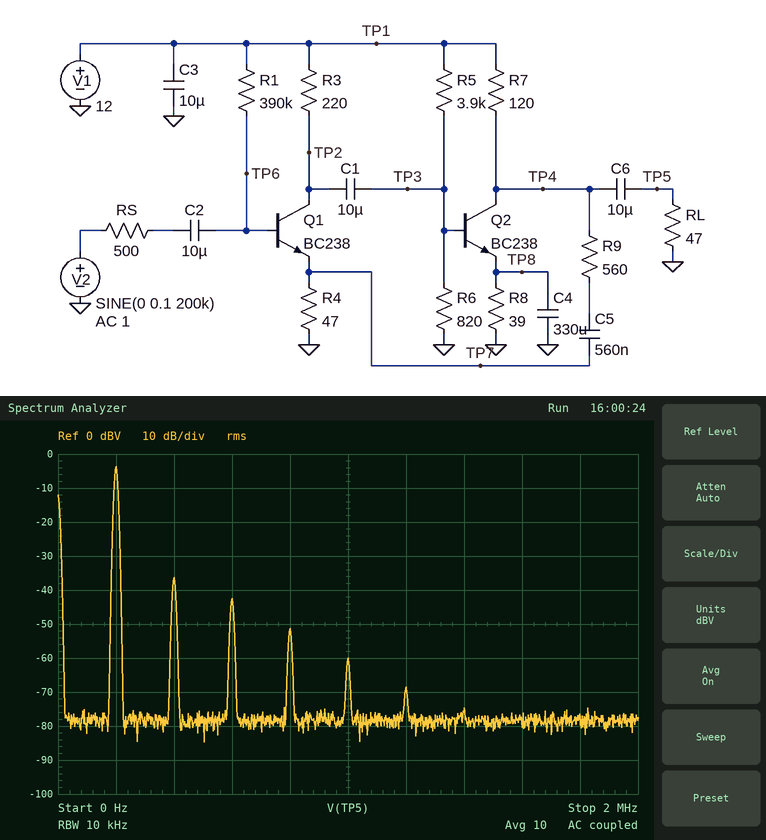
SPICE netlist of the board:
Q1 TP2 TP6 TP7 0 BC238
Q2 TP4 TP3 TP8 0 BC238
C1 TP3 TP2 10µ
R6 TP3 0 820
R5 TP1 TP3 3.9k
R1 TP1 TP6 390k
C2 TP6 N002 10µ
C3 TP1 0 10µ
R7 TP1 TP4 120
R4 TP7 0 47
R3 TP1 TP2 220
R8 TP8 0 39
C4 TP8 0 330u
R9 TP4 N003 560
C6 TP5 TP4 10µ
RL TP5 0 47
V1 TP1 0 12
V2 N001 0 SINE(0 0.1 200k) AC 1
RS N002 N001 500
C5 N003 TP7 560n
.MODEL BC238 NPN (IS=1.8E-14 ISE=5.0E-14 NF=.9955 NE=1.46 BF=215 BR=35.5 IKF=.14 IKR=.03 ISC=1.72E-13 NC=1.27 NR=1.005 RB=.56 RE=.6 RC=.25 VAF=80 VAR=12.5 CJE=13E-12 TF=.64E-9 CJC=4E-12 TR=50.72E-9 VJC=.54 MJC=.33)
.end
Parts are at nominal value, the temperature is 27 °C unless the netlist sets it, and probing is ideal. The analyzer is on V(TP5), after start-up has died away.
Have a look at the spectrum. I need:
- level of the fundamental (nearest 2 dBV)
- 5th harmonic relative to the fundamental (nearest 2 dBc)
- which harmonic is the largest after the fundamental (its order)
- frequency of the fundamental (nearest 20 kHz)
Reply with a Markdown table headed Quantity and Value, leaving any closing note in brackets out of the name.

| Quantity | Value |
|---|---|
| level of the fundamental | -4 dBV |
| 5th harmonic relative to the fundamental | -56 dBc |
| which harmonic is the largest after the fundamental | 2 |
| frequency of the fundamental | 200 kHz |
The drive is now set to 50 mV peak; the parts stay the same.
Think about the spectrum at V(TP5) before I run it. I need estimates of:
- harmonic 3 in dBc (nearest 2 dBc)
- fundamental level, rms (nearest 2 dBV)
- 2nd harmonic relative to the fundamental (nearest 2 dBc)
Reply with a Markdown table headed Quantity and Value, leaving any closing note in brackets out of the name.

| Quantity | Value |
|---|---|
| harmonic 3 in dBc | -56 dBc |
| fundamental level, rms | -10 dBV |
| 2nd harmonic relative to the fundamental | -44 dBc |
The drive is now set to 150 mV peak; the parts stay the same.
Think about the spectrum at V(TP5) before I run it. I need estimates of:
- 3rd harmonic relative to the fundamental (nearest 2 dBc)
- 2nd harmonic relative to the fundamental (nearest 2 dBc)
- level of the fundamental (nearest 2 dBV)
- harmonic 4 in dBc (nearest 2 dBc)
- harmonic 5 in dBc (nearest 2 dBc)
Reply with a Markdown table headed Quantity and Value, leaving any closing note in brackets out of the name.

| Quantity | Value |
|---|---|
| 3rd harmonic relative to the fundamental | -26 dBc |
| 2nd harmonic relative to the fundamental | -22 dBc |
| level of the fundamental | 0 dBV |
| harmonic 4 in dBc | -34 dBc |
| harmonic 5 in dBc | -44 dBc |
